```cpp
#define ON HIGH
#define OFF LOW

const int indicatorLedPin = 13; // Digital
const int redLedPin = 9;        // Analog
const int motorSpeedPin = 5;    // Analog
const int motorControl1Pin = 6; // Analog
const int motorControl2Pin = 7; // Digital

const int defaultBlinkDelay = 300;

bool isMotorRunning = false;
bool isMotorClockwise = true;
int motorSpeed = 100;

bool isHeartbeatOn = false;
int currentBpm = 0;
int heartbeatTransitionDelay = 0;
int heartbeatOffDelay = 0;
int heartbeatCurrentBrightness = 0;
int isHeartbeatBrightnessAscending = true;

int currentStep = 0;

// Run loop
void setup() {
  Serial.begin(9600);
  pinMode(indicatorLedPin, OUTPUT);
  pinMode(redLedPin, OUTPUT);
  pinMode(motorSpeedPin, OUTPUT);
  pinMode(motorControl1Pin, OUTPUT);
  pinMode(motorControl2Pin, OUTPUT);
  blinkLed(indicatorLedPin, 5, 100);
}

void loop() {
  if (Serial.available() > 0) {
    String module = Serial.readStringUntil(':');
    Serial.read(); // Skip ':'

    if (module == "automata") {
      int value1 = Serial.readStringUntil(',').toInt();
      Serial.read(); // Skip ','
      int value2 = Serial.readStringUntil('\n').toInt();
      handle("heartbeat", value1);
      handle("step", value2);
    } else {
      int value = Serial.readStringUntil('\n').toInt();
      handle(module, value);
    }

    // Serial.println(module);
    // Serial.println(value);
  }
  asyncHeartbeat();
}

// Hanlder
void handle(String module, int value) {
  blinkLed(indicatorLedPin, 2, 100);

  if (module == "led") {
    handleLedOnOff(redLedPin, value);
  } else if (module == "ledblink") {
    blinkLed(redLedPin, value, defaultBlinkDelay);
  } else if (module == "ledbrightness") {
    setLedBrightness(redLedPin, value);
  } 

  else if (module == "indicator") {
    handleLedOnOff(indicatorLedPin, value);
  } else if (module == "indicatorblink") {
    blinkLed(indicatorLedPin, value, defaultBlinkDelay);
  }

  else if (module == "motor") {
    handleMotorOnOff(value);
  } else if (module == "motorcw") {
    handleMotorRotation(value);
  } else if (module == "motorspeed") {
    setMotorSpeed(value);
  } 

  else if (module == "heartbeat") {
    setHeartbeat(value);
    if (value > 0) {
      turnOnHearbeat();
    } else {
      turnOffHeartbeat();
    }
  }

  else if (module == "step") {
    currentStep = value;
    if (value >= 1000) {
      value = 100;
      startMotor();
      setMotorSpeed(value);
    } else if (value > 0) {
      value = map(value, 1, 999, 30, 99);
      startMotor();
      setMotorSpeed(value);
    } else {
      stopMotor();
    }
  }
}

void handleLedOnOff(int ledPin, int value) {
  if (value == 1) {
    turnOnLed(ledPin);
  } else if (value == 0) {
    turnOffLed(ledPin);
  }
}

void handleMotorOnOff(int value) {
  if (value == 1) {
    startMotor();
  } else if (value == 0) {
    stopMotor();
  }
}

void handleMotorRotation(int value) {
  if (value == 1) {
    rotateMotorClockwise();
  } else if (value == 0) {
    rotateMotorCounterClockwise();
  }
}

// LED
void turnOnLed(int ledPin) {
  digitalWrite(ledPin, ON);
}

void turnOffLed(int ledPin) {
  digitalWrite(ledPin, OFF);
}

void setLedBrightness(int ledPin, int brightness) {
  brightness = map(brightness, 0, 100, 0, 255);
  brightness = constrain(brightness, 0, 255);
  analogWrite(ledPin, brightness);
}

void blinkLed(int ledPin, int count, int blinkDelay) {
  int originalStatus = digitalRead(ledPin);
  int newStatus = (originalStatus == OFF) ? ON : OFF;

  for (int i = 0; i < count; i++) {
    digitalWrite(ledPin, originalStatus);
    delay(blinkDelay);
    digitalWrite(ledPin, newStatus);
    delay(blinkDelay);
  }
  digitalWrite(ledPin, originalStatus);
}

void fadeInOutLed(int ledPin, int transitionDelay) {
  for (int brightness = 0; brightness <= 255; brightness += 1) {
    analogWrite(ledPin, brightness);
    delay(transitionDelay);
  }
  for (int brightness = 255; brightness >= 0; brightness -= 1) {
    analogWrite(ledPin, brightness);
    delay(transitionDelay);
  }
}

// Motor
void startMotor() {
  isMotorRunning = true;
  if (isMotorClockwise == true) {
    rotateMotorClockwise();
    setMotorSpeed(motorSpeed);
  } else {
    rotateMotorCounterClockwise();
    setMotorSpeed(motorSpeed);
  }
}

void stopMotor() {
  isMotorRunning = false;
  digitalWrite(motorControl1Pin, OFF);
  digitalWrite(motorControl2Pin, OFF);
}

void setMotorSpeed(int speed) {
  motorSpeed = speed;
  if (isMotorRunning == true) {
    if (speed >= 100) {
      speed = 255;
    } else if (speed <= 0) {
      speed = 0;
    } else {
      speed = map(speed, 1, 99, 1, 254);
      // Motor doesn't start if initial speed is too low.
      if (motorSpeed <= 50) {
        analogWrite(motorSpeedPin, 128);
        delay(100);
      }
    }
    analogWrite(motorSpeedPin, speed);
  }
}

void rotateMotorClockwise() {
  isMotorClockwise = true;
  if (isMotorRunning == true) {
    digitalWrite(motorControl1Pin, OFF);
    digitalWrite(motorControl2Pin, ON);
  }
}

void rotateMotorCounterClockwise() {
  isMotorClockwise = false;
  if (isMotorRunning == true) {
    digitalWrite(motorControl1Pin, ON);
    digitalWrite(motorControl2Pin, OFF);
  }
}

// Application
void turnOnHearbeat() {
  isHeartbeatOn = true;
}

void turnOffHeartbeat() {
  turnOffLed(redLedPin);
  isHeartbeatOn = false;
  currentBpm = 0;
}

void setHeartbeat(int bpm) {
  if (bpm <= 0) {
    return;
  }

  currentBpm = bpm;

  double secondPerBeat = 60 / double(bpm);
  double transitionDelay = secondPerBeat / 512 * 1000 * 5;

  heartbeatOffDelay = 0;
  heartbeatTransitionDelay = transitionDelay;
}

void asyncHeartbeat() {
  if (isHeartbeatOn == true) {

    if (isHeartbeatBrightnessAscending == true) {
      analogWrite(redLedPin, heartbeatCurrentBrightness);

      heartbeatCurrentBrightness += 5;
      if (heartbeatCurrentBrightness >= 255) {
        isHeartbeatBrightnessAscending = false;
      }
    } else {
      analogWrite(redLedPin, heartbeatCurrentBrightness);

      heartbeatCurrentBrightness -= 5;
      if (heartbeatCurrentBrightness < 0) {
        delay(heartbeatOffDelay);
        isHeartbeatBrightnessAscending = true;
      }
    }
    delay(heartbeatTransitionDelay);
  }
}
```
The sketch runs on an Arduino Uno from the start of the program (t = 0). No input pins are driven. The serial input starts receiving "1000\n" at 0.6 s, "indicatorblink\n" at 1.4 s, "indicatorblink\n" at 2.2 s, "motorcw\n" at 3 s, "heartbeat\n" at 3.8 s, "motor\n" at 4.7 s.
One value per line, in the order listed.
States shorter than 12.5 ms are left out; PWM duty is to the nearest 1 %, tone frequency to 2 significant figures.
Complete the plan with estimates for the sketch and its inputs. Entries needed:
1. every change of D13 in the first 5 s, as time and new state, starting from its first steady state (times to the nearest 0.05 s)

0 s low; 0.1 s high; 0.2 s low; 0.3 s high; 0.4 s low; 0.5 s high; 0.6 s low; 0.7 s high; 0.8 s low; 0.9 s high; 1 s low
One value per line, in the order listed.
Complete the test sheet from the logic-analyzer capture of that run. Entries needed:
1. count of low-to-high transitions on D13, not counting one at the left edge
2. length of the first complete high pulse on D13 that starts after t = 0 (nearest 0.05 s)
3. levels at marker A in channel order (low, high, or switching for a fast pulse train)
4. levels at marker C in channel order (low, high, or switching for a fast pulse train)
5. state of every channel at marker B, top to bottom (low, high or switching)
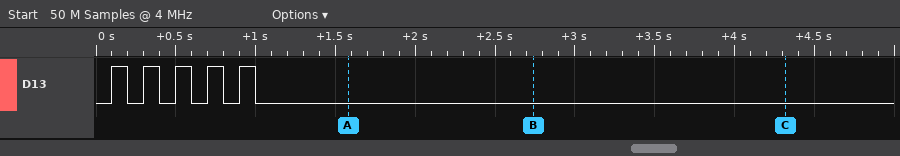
5
0.10 s
D13 low
D13 low
D13 low
